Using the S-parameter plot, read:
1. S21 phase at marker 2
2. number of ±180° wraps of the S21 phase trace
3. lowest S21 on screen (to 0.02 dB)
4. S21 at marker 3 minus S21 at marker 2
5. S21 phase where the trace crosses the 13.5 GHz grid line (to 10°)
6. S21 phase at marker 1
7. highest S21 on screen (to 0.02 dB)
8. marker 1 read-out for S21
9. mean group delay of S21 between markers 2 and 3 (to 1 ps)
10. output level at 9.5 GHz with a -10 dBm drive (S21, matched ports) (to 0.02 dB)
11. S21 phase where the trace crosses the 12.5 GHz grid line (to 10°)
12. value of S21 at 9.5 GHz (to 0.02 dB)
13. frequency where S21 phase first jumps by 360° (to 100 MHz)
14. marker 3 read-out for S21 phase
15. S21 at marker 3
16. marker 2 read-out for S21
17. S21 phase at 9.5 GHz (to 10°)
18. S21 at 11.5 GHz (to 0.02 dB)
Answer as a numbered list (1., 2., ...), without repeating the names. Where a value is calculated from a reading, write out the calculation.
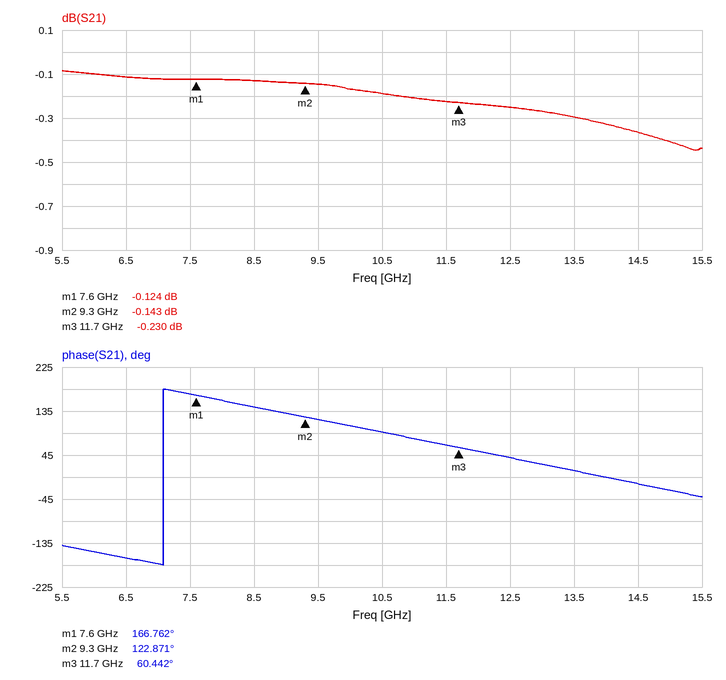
1. 122.871°
2. 1
3. -0.44 dB
4. -0.23 − (-0.143) = -0.087 dB
5. 10°
6. 166.762°
7. -0.08 dB
8. -0.124 dB
9. −(60.442° − (122.871°))/(360° × 2.4 GHz) ≈ 72 ps
10. -10 dBm + (-0.14 dB) = -10.14 dBm
11. 40°
12. -0.14 dB
13. 7.1 GHz
14. 60.442°
15. -0.230 dB
16. -0.143 dB
17. 120°
18. -0.22 dB
